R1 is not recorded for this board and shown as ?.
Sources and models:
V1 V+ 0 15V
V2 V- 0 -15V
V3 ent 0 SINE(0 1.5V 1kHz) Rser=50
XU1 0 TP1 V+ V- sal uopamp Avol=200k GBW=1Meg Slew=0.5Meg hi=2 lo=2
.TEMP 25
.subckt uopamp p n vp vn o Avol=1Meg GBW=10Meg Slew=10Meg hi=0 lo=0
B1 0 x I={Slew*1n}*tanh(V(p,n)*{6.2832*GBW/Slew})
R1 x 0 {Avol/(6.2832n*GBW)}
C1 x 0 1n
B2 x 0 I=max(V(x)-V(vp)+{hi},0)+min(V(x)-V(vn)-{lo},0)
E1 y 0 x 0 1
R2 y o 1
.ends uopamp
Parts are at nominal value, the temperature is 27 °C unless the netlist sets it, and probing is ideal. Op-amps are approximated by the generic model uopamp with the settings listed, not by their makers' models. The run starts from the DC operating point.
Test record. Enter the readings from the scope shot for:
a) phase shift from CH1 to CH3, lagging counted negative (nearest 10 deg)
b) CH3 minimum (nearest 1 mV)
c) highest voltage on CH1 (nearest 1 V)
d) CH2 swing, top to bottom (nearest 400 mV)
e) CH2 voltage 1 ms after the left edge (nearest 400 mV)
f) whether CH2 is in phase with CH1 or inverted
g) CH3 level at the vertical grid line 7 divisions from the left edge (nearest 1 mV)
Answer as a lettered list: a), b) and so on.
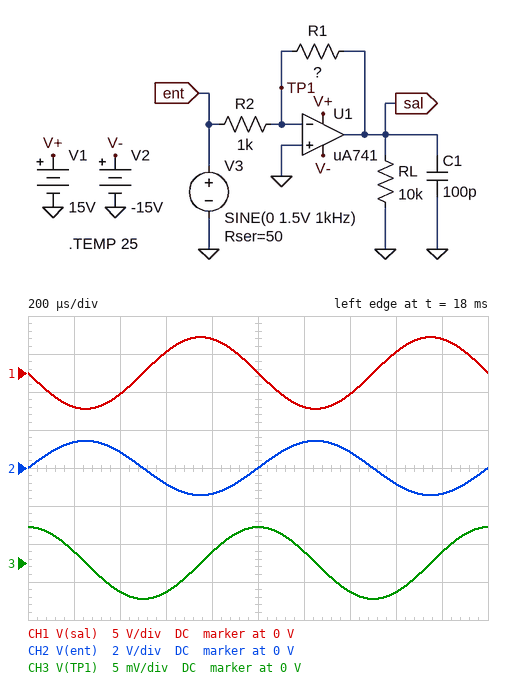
a) -90 deg
b) -5 mV
c) 5 V
d) 2.8 V
e) 0 V
f) inverted
g) -4 mV
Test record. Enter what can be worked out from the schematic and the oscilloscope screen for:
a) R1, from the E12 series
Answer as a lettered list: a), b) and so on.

a) 3.3 kΩ
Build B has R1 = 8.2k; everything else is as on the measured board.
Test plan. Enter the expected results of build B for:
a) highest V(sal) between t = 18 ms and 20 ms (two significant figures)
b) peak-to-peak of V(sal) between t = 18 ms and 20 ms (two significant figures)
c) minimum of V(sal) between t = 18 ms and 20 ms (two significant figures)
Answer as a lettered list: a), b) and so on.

a) 12 V
b) 23 V
c) -12 V
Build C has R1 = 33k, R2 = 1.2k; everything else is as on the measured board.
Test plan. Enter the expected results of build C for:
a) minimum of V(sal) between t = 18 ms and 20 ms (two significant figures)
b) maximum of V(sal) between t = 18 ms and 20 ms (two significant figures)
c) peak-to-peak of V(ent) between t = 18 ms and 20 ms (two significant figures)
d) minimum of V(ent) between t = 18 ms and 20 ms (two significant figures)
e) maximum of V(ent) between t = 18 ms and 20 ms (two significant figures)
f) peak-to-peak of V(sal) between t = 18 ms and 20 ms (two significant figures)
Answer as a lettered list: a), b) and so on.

a) -13 V
b) 13 V
c) 3.0 V
d) -1.5 V
e) 1.5 V
f) 26 V
